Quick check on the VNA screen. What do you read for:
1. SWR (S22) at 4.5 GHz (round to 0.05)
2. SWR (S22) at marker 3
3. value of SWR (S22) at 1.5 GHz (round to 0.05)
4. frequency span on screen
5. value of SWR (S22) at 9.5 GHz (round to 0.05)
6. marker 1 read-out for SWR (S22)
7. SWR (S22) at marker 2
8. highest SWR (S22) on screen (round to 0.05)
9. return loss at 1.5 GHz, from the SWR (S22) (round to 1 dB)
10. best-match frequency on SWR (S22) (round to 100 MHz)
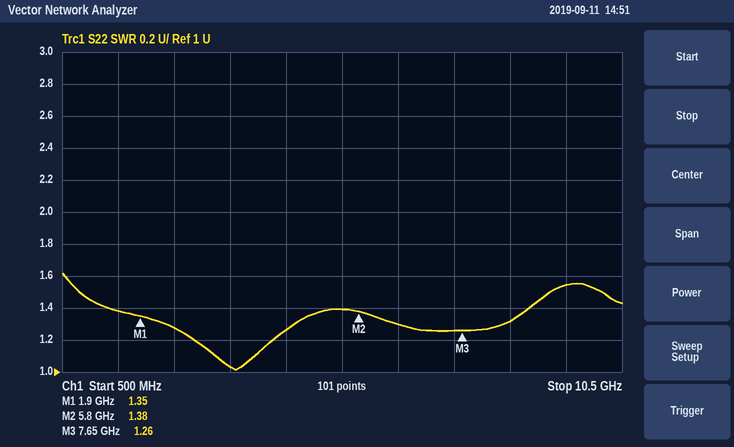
1.25
1.26
1.40
10 GHz
1.55
1.35
1.38
1.60
16 dB
3.6 GHz
